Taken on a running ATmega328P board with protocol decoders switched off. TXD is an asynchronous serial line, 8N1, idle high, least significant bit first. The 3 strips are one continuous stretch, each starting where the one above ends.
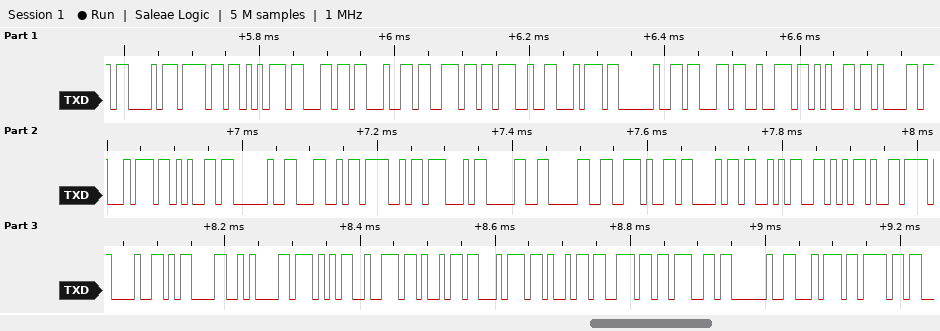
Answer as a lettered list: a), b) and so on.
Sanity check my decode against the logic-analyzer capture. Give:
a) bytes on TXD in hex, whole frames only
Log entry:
a) 43 6F 75 6C 64 6E 27 74 20 63 72 65 61 74 65 20 4C 4F 47 30 30 2E 43 53 56 D9 21 0D 0A 57 72 69 74 69 6E 67 20 74 6F
